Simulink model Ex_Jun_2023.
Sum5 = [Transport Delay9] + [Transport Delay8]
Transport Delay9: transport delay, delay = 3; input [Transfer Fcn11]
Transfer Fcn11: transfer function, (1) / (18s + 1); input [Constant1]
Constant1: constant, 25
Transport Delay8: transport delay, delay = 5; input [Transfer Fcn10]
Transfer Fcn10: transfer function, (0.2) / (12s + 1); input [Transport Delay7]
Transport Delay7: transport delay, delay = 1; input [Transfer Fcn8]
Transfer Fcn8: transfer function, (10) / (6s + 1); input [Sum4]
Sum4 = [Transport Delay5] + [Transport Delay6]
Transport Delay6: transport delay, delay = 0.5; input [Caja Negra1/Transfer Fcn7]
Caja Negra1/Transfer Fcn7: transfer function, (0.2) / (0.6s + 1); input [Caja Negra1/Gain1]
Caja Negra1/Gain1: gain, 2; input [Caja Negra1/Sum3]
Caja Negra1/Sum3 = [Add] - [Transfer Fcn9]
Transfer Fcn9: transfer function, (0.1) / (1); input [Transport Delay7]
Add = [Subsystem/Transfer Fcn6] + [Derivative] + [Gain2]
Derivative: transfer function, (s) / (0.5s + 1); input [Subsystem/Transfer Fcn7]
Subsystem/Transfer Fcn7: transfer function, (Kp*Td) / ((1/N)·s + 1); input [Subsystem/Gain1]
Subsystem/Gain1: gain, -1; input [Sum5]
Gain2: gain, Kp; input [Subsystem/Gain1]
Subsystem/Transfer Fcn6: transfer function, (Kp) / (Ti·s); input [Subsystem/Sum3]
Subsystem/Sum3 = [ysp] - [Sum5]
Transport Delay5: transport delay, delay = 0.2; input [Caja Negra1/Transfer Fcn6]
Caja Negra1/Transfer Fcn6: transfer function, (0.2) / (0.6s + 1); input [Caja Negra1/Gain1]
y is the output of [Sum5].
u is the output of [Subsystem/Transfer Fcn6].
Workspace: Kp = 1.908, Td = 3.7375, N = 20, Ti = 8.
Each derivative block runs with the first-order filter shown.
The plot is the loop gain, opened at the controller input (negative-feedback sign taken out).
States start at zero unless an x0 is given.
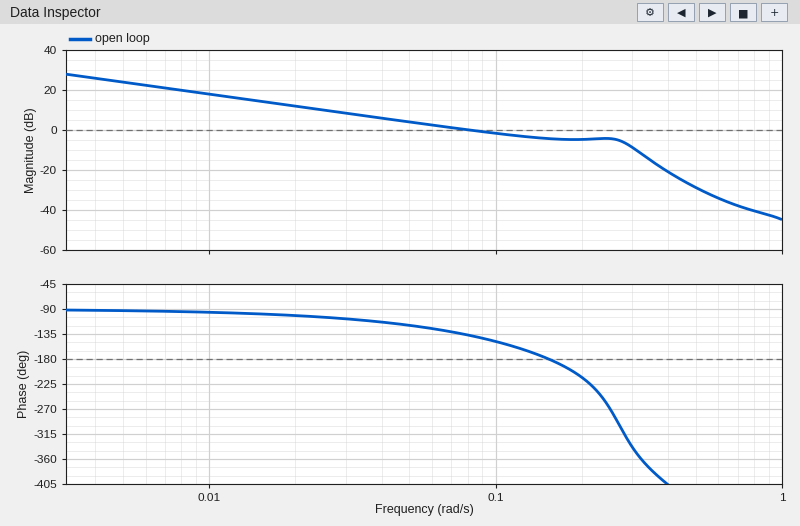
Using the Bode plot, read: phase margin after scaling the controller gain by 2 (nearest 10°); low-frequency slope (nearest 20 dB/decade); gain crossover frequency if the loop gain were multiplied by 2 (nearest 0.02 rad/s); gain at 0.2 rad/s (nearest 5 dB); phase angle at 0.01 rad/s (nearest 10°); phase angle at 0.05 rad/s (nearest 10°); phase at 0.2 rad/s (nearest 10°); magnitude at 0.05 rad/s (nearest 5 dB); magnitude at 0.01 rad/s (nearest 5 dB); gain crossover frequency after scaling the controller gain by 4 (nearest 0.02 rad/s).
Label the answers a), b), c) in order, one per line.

a) -130°
b) -20 dB/decade
c) 0.28 rad/s
d) -5 dB
e) -100°
f) -120°
g) -210°
h) 5 dB
i) 20 dB
j) 0.32 rad/s
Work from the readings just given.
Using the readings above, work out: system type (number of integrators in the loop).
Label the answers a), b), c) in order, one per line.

a) 1
